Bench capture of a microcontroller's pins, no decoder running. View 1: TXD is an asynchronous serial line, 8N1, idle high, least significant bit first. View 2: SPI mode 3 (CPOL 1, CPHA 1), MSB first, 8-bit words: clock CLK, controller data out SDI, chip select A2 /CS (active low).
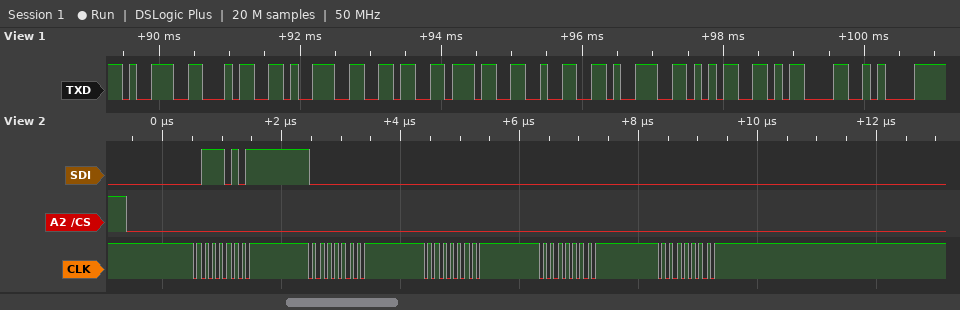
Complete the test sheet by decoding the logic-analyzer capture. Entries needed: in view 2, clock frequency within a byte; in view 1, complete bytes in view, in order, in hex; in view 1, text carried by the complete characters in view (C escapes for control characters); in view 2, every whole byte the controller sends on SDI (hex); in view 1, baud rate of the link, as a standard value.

8 MHz
0x39 0x34 0x39 0x36 0x37 0x32 0x39 0x35 0x0D 0x0A
"94967295\r\n"
75 00 00 00 00
9600 baud
